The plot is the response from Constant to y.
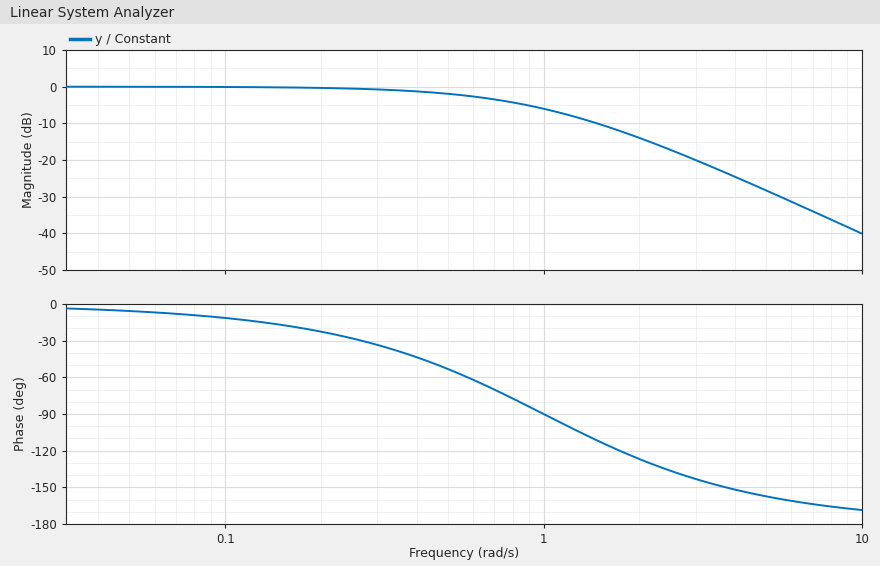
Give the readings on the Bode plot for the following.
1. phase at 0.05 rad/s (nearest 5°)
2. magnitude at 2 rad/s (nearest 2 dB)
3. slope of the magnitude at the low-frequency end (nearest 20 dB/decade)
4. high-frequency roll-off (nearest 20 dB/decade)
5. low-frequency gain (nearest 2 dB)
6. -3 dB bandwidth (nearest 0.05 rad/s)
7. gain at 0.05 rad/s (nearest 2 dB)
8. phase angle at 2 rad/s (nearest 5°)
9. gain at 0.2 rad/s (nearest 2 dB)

-5°
-14 dB
0 dB/decade
-40 dB/decade
0 dB
0.65 rad/s
0 dB
-125°
0 dB
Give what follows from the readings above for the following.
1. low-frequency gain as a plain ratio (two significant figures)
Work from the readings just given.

1.0
